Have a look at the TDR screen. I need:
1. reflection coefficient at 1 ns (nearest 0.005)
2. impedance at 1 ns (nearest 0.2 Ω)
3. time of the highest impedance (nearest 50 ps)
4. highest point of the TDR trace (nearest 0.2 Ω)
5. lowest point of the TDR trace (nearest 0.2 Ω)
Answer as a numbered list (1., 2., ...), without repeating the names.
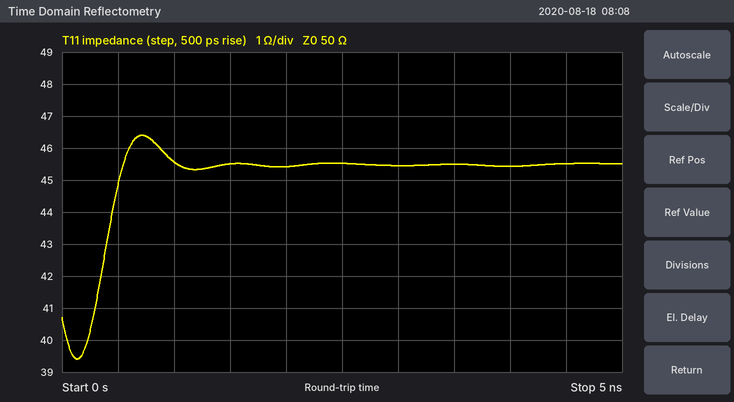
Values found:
1. -0.045
2. 45.6 Ω
3. 700 ps
4. 46.4 Ω
5. 39.4 Ω
